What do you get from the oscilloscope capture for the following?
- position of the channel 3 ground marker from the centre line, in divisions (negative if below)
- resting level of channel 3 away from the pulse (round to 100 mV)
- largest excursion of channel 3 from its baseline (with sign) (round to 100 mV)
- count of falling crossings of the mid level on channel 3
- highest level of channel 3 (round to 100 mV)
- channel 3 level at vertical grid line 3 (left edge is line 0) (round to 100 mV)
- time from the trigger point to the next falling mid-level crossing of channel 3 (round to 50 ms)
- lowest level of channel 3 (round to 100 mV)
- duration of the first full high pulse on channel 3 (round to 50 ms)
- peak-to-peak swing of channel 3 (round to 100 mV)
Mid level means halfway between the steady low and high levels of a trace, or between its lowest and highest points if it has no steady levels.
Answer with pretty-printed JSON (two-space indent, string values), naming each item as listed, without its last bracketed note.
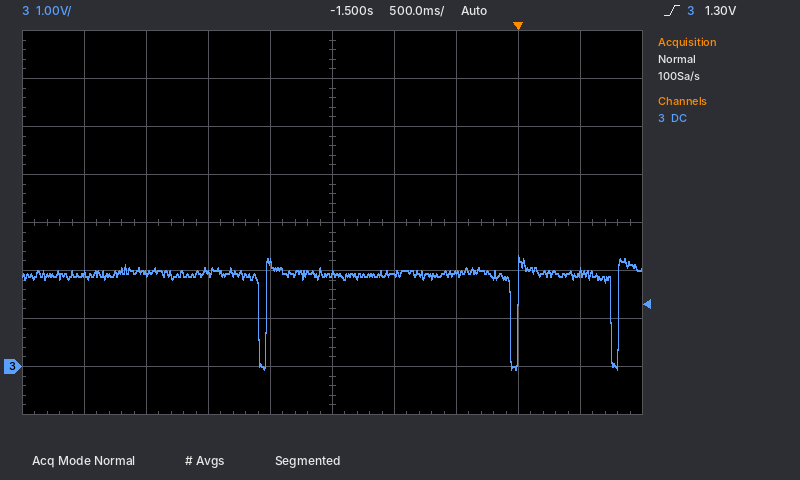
{
  "position of the channel 3 ground marker from the centre line, in divisions": "-3.0 div",
  "resting level of channel 3 away from the pulse": "1.9 V",
  "largest excursion of channel 3 from its baseline (with sign)": "-2.0 V",
  "count of falling crossings of the mid level on channel 3": "3",
  "highest level of channel 3": "2.3 V",
  "channel 3 level at vertical grid line 3 (left edge is line 0)": "2.0 V",
  "time from the trigger point to the next falling mid-level crossing of channel 3": "750 ms",
  "lowest level of channel 3": "-100 mV",
  "duration of the first full high pulse on channel 3": "1.95 s",
  "peak-to-peak swing of channel 3": "2.4 V"
}
